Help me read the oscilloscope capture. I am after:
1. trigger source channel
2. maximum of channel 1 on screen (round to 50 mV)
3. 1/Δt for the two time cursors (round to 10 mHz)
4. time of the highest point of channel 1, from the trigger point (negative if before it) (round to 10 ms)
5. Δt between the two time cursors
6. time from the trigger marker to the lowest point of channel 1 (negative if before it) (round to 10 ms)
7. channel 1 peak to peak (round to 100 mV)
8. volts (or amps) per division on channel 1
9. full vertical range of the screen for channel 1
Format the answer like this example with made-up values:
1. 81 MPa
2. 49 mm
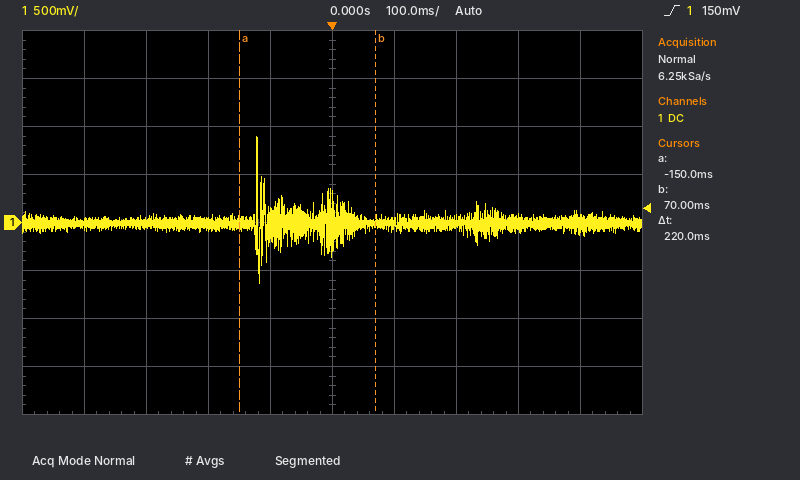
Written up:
1. channel 1
2. 900 mV
3. 4.55 Hz
4. -120 ms
5. 220 ms
6. -120 ms
7. 1.50 V
8. 500 mV
9. 4 V
